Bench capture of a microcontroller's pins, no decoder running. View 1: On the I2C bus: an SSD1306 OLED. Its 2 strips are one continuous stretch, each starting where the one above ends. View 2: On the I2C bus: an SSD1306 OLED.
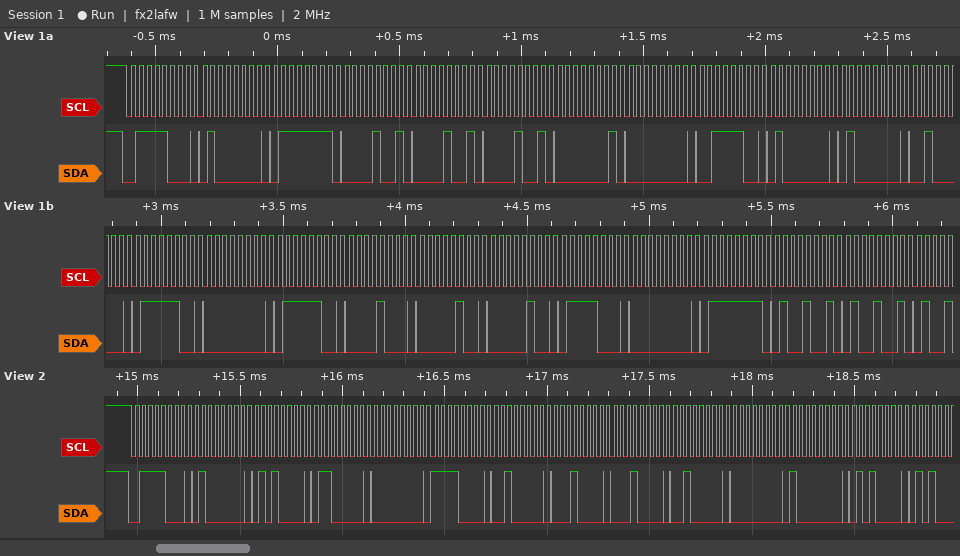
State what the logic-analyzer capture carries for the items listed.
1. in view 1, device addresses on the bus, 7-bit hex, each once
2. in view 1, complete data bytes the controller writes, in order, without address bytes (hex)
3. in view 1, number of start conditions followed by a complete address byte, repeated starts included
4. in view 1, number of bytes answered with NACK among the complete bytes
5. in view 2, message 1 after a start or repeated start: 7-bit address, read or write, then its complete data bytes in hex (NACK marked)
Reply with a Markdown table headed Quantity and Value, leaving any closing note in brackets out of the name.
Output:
| Quantity | Value |
|---|---|
| in view 1, device addresses on the bus, 7-bit hex, each once | 0x3C |
| in view 1, complete data bytes the controller writes, in order, without address bytes | 40 7F 09 09 09 01 00 3C 40 40 20 7C 00 7C 08 04 04 78 00 7F 49 49 |
| in view 1, number of start conditions followed by a complete address byte, repeated starts included | 1 |
| in view 1, number of bytes answered with NACK among the complete bytes | 0 |
| in view 2, message 1 after a start or repeated start: 7-bit address, read or write, then its complete data bytes in hex | 0x3C write: 40 50 60 00 F0 20 10 10 20 00 80 50 |
